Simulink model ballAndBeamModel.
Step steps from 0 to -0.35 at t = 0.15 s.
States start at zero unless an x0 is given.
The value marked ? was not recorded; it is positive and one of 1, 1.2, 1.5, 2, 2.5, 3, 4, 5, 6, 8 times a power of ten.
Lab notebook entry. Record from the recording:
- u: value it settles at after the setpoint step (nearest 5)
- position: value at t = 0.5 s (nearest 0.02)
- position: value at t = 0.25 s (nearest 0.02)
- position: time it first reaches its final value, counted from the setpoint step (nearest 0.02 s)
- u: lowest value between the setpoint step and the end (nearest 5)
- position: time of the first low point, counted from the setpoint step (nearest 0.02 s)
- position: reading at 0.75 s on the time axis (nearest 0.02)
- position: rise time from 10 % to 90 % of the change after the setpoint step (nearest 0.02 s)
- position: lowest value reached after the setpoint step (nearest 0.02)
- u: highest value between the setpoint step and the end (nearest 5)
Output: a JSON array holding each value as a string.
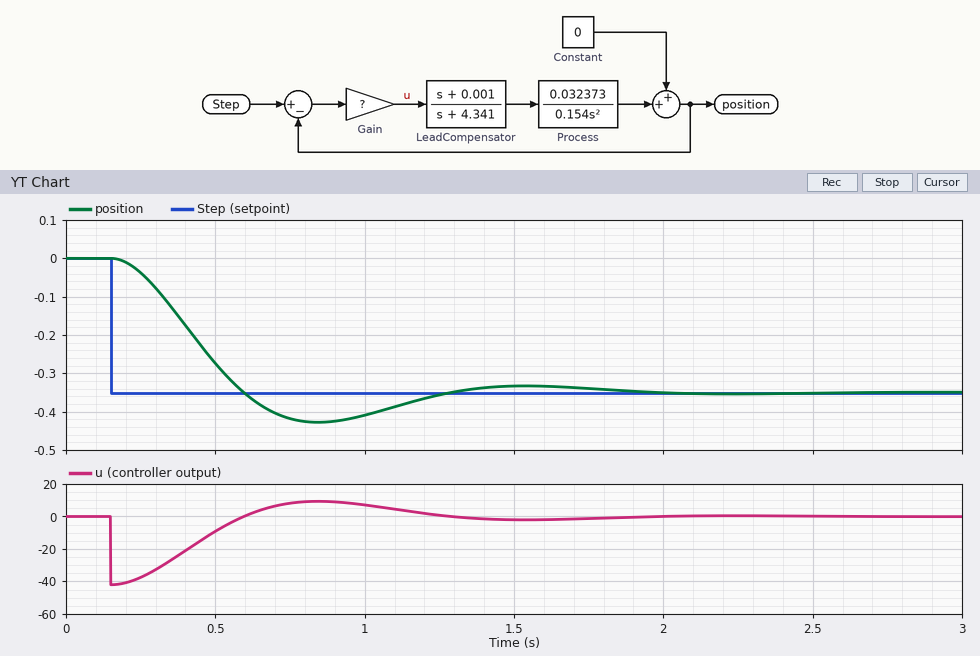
["0", "-0.28", "-0.04", "0.44 s", "-40", "0.70 s", "-0.42", "0.30 s", "-0.42", "10"]
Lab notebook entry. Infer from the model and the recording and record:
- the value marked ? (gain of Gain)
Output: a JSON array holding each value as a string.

["120"]
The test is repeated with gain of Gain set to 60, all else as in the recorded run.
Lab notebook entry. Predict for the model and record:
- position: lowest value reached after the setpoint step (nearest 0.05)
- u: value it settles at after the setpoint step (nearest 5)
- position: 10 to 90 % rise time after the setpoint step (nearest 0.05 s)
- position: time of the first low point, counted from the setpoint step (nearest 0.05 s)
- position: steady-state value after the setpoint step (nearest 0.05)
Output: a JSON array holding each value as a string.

["-0.40", "0", "0.55 s", "1.10 s", "-0.35"]
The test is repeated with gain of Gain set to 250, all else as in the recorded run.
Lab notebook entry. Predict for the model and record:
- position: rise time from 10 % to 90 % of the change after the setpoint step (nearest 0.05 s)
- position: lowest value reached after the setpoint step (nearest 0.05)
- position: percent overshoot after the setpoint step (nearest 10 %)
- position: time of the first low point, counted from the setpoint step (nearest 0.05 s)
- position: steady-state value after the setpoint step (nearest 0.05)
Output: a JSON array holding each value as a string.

["0.20 s", "-0.50", "40 %", "0.45 s", "-0.35"]
